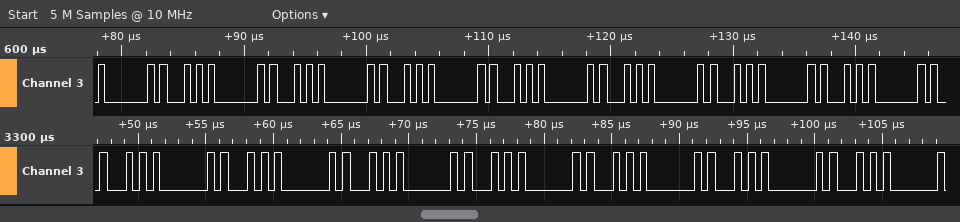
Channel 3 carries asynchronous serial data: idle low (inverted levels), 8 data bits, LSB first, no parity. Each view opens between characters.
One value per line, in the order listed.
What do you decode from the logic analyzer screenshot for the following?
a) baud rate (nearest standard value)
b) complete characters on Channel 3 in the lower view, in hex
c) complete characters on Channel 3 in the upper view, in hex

2000000 baud
57, 5D, 7F, 57, 5D, 7F, 57, 5D, 7F, 57
7F, 57, 5D, 7F, 57, 5D, 7F, 57, 5D, 7F, 57
